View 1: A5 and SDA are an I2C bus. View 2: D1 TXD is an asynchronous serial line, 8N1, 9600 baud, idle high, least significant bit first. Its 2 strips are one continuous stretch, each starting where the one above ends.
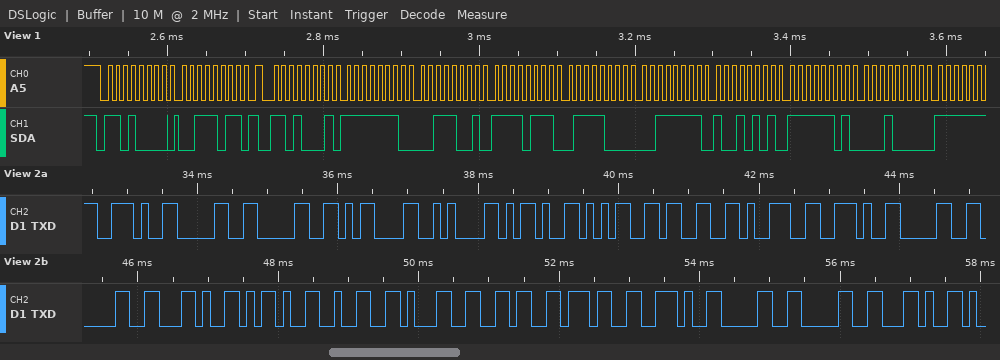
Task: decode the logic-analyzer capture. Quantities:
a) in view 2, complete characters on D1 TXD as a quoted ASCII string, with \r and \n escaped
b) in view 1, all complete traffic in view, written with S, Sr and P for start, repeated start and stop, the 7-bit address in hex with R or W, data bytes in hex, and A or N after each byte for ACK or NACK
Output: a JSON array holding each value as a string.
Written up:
["\".00\\r\\n-539.00,-2167.00,\"", "S 68W A 3B A Sr 68R A FE A 39 A F7 A 78 A 3F A 95 A FD A 10 A"]
